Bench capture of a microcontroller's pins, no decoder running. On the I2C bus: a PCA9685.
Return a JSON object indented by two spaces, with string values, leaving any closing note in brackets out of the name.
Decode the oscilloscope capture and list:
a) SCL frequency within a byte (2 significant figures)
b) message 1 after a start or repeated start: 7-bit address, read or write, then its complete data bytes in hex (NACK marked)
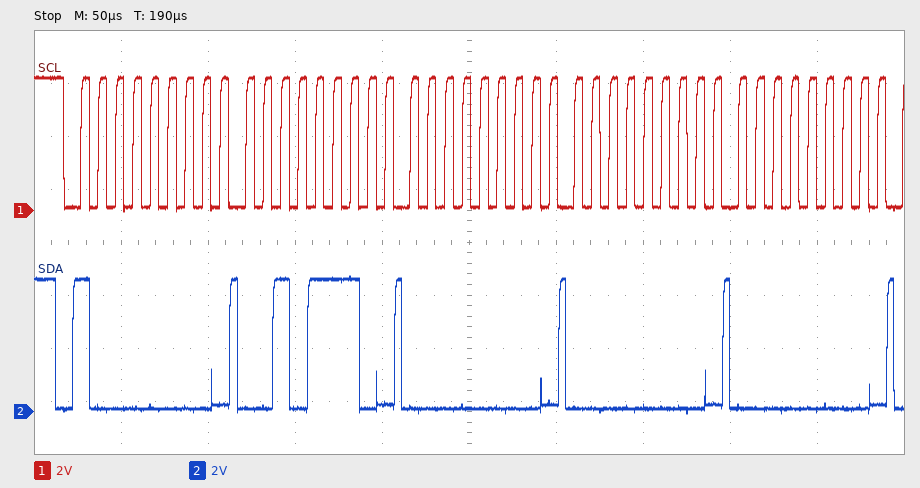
{
  "SCL frequency within a byte": "100 kHz",
  "message 1 after a start or repeated start: 7-bit address, read or write, then its complete data bytes in hex": "0x40 write: 2E 00 00 00"
}
